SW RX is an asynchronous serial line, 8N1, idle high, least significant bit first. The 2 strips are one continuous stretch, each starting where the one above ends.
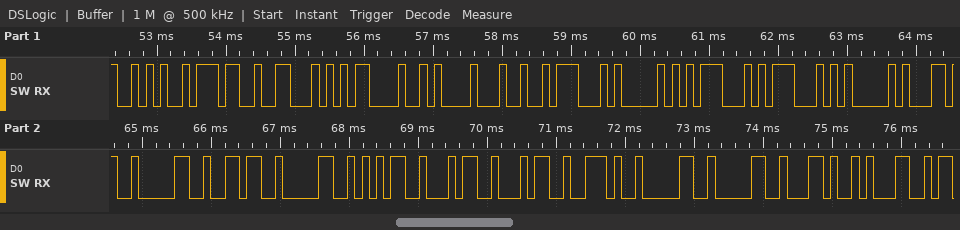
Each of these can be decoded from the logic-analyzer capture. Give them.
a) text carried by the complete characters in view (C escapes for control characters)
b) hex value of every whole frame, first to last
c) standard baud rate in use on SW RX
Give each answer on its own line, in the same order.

"*7F\r\n$GPGGA,060544.00,1"
0x2A 0x37 0x46 0x0D 0x0A 0x24 0x47 0x50 0x47 0x47 0x41 0x2C 0x30 0x36 0x30 0x35 0x34 0x34 0x2E 0x30 0x30 0x2C 0x31
9600 baud
